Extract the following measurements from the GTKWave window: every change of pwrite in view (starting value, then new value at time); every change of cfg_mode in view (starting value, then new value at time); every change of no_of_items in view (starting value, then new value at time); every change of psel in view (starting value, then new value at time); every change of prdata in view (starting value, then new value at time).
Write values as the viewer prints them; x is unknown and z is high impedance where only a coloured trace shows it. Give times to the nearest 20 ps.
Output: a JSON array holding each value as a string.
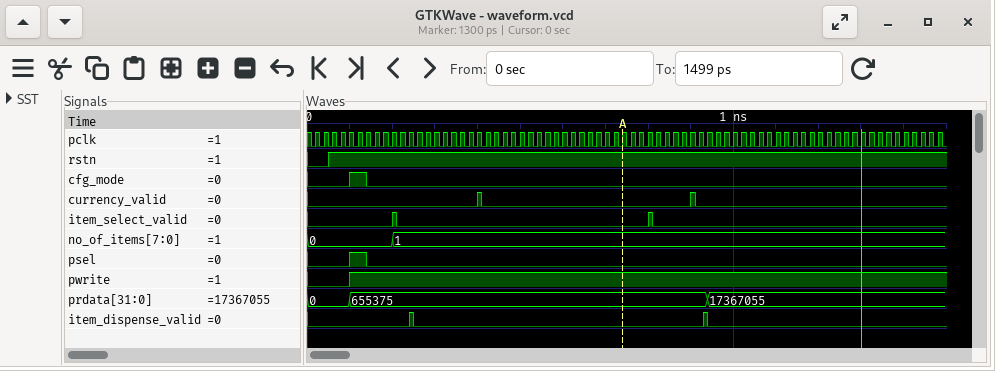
["0, 1 at 100 ps", "0, 1 at 100 ps, 0 at 140 ps", "0, 1 at 200 ps", "0, 1 at 100 ps, 0 at 140 ps", "0, 655375 at 100 ps, 17367055 at 940 ps"]
